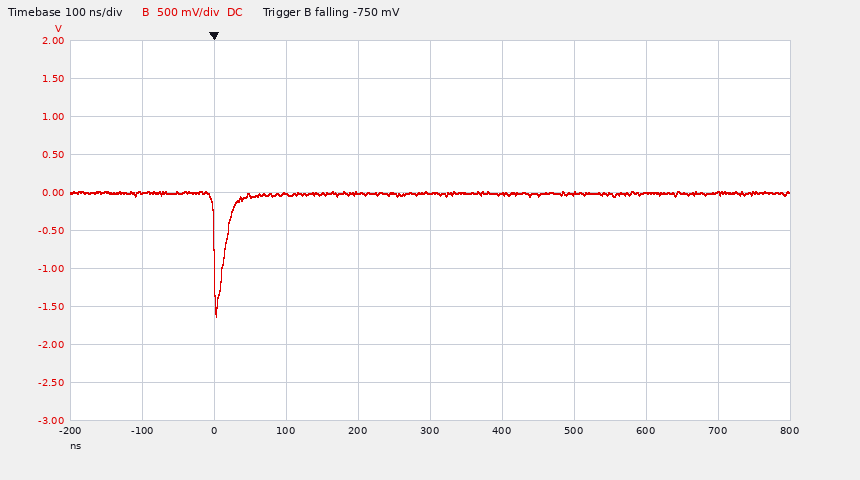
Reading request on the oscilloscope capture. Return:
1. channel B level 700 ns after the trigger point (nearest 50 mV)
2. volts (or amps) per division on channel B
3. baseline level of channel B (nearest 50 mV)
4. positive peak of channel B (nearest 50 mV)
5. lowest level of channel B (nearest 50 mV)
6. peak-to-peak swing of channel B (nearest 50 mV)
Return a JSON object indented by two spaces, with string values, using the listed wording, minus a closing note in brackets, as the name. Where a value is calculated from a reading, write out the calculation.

{
  "channel B level 700 ns after the trigger point": "0 mV",
  "volts (or amps) per division on channel B": "500 mV",
  "baseline level of channel B": "0 mV",
  "positive peak of channel B": "0 mV",
  "lowest level of channel B": "-1.65 V",
  "peak-to-peak swing of channel B": "0 mV − (-1.65 V) = 1.65 V"
}
